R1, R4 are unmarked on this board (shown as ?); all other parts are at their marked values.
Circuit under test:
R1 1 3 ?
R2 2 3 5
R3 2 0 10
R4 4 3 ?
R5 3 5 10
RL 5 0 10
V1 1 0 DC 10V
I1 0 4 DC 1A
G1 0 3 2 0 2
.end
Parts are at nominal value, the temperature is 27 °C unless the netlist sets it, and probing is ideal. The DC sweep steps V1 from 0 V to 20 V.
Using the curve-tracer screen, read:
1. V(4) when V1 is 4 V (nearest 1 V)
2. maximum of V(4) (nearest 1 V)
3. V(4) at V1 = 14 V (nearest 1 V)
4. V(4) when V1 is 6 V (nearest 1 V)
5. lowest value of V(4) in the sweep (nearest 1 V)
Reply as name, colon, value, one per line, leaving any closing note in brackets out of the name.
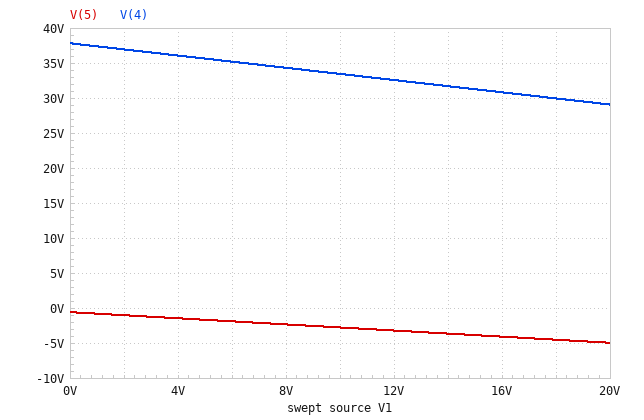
V(4) when V1 is 4 V: 36 V
maximum of V(4): 38 V
V(4) at V1 = 14 V: 32 V
V(4) when V1 is 6 V: 35 V
lowest value of V(4) in the sweep: 29 V
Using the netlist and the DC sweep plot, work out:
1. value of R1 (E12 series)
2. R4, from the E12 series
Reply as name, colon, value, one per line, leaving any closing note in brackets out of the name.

value of R1: 2.7 Ω
R4, from the E12 series: 39 Ω
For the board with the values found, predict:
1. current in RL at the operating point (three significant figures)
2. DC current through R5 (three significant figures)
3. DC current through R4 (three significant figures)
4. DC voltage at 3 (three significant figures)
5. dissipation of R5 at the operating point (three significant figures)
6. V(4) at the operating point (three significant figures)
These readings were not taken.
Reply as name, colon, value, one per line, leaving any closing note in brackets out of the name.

current in RL at the operating point: 278 mA
DC current through R5: 278 mA
DC current through R4: 1.00 A
DC voltage at 3: -5.56 V
dissipation of R5 at the operating point: 772 mW
V(4) at the operating point: 33.4 V
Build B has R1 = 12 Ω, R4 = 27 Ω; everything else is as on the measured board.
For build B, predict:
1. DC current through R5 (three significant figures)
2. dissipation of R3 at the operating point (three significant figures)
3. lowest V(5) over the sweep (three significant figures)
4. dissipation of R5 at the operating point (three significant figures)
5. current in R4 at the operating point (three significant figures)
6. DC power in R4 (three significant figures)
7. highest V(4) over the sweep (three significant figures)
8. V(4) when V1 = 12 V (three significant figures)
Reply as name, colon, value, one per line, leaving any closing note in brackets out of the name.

DC current through R5: 80.9 mA
dissipation of R3 at the operating point: 116 mW
lowest V(5) over the sweep: -1.18 V
dissipation of R5 at the operating point: 65.4 mW
current in R4 at the operating point: 1.00 A
DC power in R4: 27.0 W
highest V(4) over the sweep: 26.1 V
V(4) when V1 = 12 V: 25.2 V
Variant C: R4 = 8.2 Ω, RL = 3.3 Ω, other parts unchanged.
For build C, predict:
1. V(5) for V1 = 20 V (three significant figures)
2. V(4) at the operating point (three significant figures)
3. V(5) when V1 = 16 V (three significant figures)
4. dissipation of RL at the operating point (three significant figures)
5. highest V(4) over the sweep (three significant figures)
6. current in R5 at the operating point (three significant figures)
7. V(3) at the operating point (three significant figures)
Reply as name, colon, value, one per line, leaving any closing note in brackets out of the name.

V(5) for V1 = 20 V: -2.54 V
V(4) at the operating point: 2.47 V
V(5) when V1 = 16 V: -2.09 V
dissipation of RL at the operating point: 612 mW
highest V(4) over the sweep: 6.98 V
current in R5 at the operating point: 431 mA
V(3) at the operating point: -5.73 V
